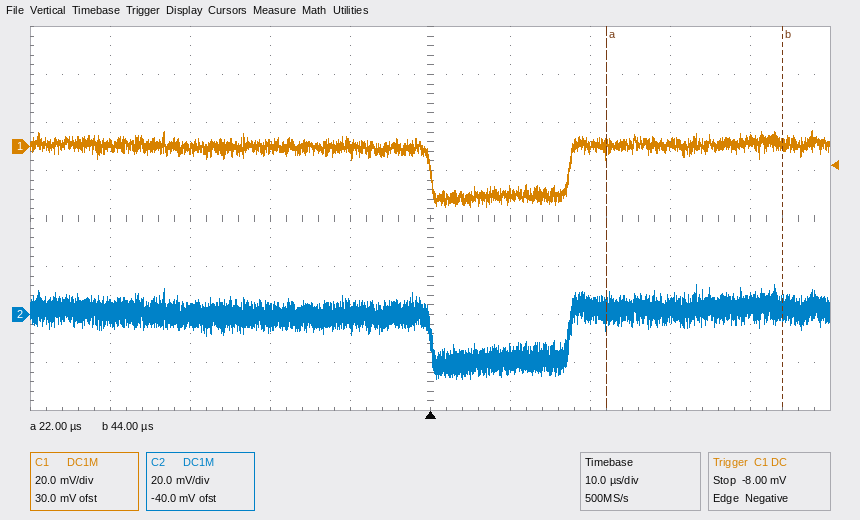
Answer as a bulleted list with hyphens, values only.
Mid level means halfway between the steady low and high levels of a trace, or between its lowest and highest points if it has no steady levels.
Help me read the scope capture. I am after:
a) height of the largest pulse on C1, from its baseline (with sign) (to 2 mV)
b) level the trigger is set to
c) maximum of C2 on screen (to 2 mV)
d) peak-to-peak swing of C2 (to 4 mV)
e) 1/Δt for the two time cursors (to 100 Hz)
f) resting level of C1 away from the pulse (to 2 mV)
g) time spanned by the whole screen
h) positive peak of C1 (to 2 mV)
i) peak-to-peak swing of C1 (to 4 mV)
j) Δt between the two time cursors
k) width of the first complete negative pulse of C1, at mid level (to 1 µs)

- -26 mV
- -8.00 mV
- 12 mV
- 40 mV
- 45.5 kHz
- 0 mV
- 100 µs
- 6 mV
- 32 mV
- 22 µs
- 17 µs
